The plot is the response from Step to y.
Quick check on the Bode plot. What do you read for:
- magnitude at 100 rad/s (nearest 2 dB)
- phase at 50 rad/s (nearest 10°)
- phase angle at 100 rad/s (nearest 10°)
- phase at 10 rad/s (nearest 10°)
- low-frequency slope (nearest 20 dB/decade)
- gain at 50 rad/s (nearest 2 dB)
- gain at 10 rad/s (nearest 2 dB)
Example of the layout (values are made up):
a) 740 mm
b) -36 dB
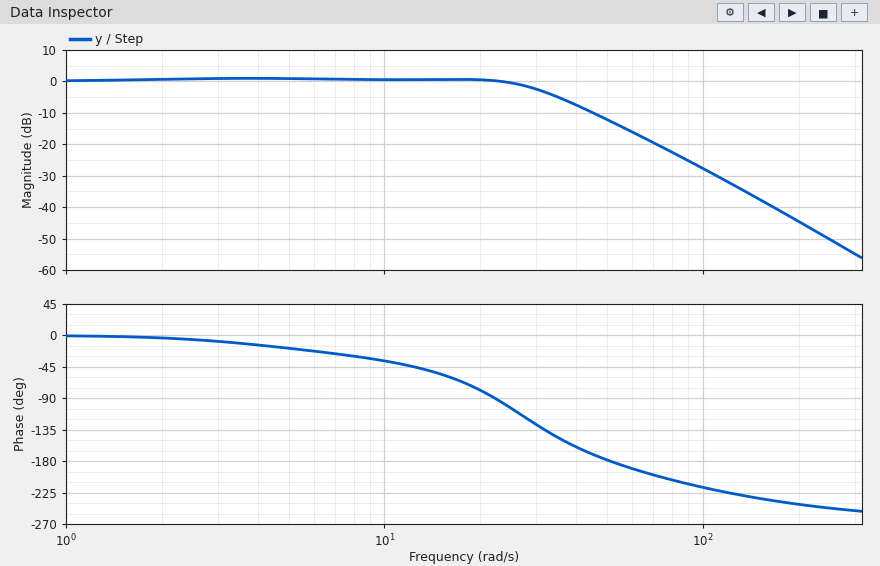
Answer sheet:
a) -28 dB
b) -180°
c) -220°
d) -40°
e) 0 dB/decade
f) -12 dB
g) 0 dB
